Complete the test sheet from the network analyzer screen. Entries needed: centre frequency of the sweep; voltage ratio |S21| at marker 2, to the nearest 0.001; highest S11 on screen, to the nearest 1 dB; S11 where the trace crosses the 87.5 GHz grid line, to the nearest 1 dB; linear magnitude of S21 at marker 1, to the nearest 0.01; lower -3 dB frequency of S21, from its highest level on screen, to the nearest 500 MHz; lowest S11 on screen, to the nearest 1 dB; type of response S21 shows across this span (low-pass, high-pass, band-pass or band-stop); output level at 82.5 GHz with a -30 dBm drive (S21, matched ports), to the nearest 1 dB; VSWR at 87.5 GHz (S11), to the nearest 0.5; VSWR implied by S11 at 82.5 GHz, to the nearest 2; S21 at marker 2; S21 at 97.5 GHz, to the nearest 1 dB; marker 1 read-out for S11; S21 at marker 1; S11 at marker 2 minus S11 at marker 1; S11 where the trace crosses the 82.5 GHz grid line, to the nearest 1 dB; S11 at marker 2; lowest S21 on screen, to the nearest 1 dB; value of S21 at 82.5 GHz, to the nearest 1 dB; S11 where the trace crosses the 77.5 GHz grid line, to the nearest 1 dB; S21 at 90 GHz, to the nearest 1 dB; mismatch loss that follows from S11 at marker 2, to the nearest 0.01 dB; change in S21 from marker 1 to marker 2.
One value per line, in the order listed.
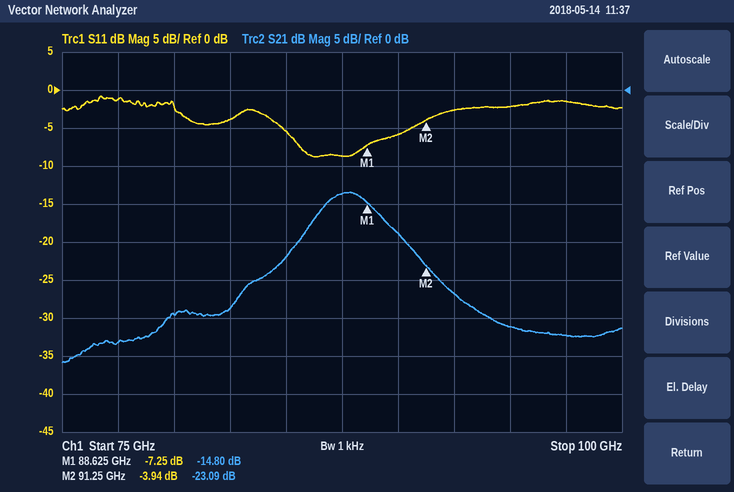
87.5 GHz
0.070
-1 dB
-9 dB
0.18
86.5 GHz
-9 dB
band-pass
-59 dBm
2.0
4
-23.09 dB
-32 dB
-7.25 dB
-14.80 dB
3.31 dB
-4 dB
-3.94 dB
-36 dB
-29 dB
-1 dB
-19 dB
2.24 dB
-8.29 dB
